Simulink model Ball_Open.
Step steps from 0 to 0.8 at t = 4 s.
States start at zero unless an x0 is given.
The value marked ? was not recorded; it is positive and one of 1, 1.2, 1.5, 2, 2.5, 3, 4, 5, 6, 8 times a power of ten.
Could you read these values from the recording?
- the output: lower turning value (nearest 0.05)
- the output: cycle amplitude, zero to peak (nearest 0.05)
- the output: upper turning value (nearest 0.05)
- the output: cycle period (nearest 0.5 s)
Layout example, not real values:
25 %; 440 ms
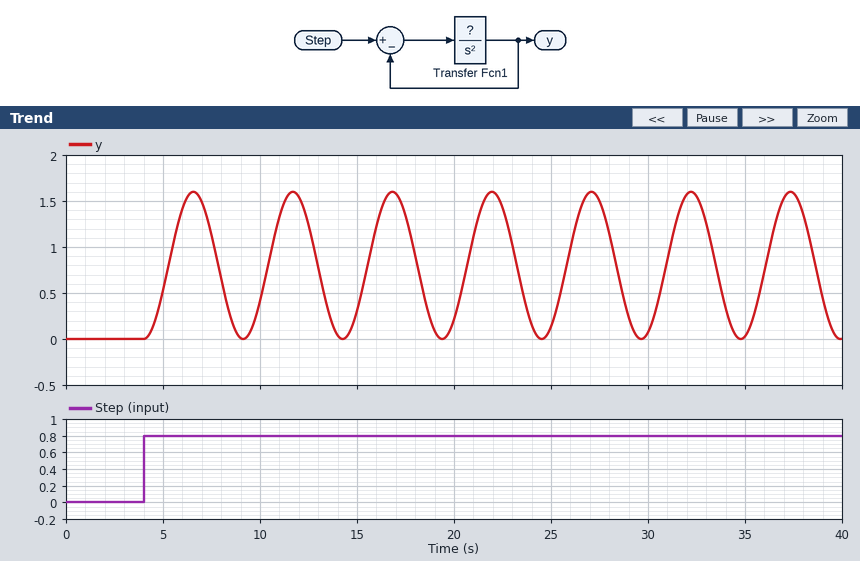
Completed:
0.00; 0.80; 1.60; 5.0 s
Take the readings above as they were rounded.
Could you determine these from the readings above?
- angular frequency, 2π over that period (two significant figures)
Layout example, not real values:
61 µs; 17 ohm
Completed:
1.3 rad/s
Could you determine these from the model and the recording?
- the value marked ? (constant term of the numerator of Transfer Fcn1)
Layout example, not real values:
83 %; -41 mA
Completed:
1.5
